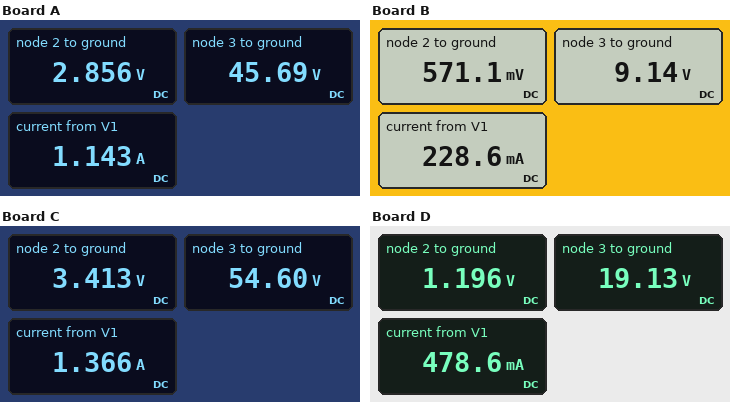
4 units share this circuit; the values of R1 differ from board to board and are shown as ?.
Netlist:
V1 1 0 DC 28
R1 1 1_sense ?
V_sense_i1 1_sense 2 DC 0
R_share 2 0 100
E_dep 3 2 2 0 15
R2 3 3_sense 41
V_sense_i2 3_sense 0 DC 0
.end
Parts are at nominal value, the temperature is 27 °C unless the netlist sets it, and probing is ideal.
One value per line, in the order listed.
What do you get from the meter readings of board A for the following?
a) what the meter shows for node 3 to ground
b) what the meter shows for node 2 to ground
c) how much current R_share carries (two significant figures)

45.69 V
2.856 V
29 mA
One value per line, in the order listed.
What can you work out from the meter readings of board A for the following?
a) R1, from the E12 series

22 Ω
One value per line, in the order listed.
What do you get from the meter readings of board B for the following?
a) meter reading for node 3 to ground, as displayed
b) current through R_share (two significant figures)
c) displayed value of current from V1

9.14 V
5.7 mA
228.6 mA
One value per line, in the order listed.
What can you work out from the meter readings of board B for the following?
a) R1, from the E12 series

120 Ω
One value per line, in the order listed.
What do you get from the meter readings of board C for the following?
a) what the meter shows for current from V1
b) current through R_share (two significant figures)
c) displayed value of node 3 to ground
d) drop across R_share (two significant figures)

1.366 A
34 mA
54.60 V
3.4 V
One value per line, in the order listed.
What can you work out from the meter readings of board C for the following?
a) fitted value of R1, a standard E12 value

18 Ω
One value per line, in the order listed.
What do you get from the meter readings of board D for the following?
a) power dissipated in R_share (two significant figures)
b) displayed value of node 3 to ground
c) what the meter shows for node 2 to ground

14 mW
19.13 V
1.196 V
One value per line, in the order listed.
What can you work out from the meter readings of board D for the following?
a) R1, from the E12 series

56 Ω
